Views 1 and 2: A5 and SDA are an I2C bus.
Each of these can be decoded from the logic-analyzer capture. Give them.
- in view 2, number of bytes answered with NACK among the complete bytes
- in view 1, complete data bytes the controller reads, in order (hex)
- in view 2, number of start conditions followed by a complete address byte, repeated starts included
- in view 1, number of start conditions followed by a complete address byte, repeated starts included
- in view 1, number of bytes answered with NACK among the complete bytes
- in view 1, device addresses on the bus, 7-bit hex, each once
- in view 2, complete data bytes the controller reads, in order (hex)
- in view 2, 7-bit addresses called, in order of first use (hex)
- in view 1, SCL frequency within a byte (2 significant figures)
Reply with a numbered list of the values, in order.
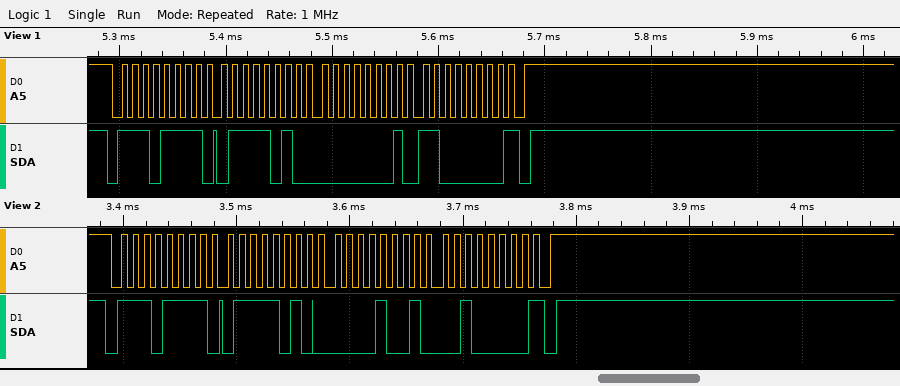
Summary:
1. 1
2. 7A 01 C0
3. 1
4. 1
5. 1
6. 0x77
7. 7A 09 20
8. 0x77
9. 100 kHz
